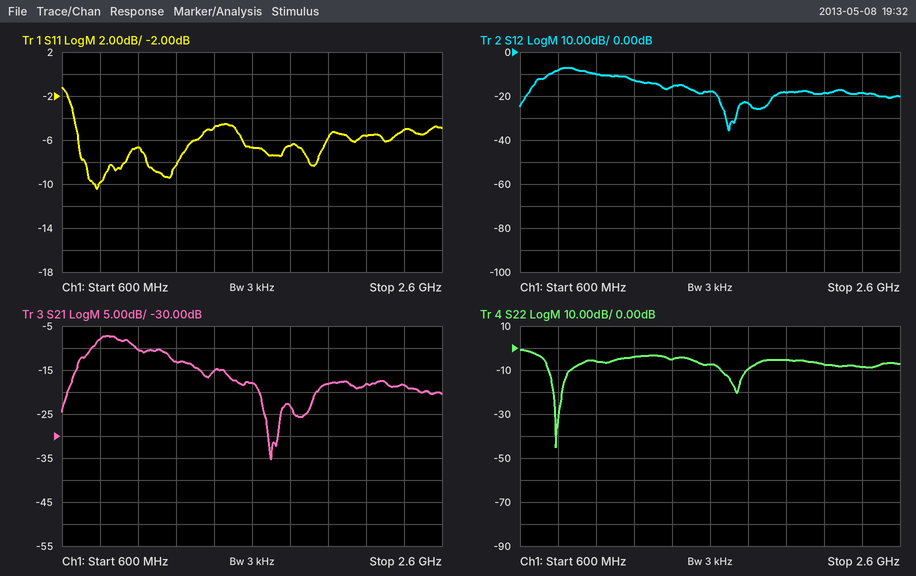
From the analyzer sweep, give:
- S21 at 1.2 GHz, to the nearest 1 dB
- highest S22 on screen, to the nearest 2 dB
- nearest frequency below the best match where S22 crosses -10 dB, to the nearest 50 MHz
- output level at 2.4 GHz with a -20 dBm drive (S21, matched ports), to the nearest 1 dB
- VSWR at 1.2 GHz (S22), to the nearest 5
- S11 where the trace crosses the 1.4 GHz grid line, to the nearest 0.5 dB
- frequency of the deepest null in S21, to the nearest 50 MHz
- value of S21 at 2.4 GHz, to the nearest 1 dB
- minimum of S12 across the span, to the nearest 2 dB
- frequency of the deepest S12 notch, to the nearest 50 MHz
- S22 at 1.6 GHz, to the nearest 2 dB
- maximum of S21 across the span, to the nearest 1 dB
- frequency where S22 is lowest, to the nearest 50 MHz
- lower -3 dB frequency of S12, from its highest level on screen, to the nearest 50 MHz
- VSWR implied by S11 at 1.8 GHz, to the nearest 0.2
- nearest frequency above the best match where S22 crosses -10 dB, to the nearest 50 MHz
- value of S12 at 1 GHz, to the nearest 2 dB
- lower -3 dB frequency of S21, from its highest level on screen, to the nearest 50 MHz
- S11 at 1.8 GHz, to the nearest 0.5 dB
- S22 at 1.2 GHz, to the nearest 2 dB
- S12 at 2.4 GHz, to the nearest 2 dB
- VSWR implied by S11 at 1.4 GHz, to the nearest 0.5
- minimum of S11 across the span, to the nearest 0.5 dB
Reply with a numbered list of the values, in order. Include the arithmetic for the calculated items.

1. -13 dB
2. 0 dB
3. 750 MHz
4. -20 dBm + (-18 dB) = -38 dBm
5. |Γ| = 10^(-4/20) = 0.6310; VSWR = (1 + 0.6310)/(1 − 0.6310) ≈ 4.42, so 5 to the nearest 5
6. -5.0 dB
7. 1.70 GHz
8. -18 dB
9. -36 dB
10. 1.70 GHz
11. -8 dB
12. -7 dB
13. 800 MHz
14. 750 MHz
15. |Γ| = 10^(-6.5/20) = 0.4732; VSWR = (1 + 0.4732)/(1 − 0.4732) ≈ 2.8
16. 850 MHz
17. -10 dB
18. 750 MHz
19. -6.5 dB
20. -4 dB
21. -18 dB
22. |Γ| = 10^(-5/20) = 0.5623; VSWR = (1 + 0.5623)/(1 − 0.5623) ≈ 3.57, so 3.5 to the nearest 0.5
23. -10.5 dB
